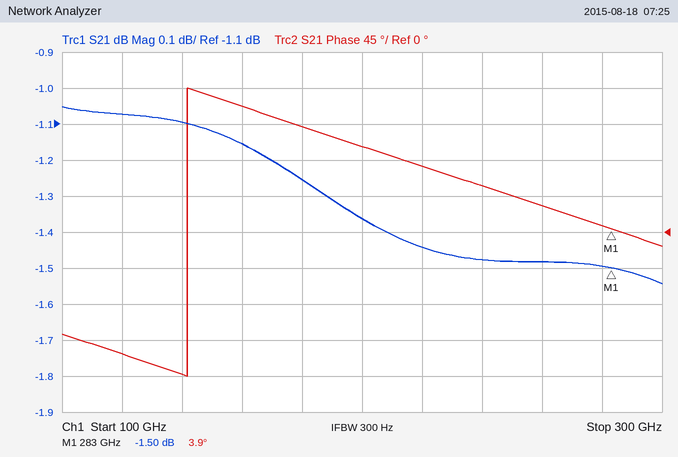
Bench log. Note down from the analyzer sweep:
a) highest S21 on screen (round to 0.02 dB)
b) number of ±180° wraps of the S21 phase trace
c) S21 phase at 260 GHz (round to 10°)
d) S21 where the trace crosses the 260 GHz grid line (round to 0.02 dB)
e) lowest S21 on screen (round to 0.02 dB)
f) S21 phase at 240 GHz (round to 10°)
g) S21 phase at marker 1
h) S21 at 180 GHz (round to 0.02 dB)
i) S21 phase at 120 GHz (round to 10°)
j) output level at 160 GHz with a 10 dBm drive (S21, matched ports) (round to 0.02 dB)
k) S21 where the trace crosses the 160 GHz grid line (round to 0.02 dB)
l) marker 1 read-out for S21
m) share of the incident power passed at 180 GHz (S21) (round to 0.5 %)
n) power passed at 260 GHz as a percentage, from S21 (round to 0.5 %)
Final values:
-1.06 dB
1
30°
-1.48 dB
-1.54 dB
60°
3.9°
-1.26 dB
-150°
8.84 dBm
-1.16 dB
-1.50 dB
75.0 %
71.0 %
